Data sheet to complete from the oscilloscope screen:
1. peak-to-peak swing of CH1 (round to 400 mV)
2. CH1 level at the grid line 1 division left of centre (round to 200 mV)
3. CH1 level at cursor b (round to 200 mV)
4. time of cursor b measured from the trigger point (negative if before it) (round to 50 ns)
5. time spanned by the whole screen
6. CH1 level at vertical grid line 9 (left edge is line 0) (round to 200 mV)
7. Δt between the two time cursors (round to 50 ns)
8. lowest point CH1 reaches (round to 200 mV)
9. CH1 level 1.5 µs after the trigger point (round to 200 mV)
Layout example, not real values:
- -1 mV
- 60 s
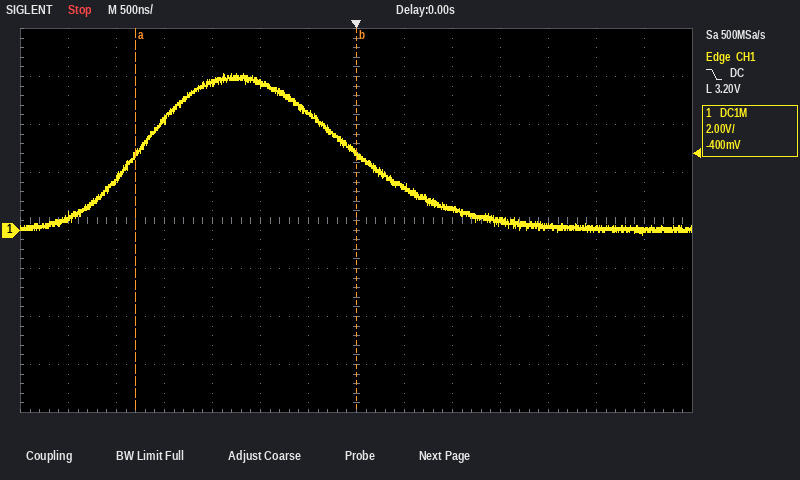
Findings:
- 6.8 V
- 4.8 V
- 3.2 V
- 0 ns
- 7 µs
- 800 mV
- 2.30 µs
- -200 mV
- 400 mV
